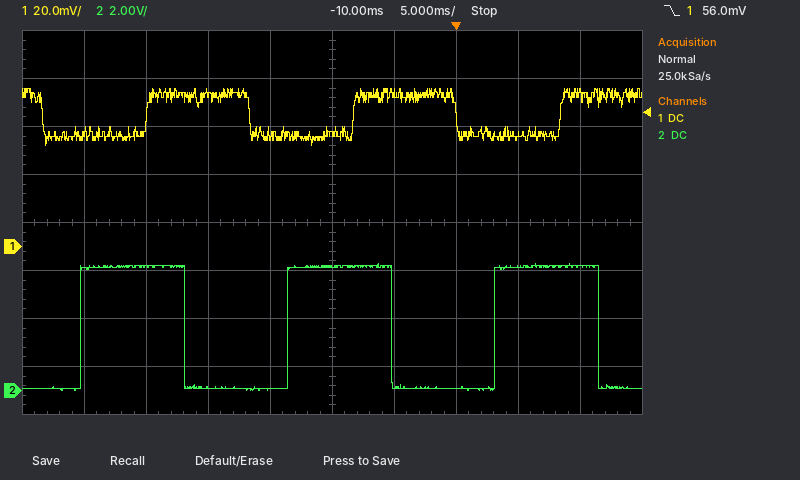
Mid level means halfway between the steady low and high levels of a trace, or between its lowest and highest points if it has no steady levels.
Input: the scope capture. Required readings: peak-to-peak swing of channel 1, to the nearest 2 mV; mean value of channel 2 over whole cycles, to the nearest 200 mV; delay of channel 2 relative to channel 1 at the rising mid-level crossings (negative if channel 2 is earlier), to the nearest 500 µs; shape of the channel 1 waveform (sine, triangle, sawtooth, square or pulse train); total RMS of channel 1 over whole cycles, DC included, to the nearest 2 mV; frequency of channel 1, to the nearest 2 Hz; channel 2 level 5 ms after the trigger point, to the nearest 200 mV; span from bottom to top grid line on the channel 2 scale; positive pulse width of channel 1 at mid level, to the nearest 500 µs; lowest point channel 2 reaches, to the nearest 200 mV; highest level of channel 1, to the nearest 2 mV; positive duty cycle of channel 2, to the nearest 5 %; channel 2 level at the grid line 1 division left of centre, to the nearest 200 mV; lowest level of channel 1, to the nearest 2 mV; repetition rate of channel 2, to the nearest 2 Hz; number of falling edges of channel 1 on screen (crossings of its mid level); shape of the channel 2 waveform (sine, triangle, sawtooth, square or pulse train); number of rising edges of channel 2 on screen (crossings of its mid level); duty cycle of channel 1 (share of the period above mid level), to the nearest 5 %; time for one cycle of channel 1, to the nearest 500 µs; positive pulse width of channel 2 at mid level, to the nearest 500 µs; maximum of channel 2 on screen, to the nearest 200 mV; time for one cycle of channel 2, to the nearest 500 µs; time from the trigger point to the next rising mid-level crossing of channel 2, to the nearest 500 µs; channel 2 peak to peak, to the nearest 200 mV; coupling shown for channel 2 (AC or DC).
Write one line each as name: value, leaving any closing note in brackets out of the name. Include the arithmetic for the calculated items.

peak-to-peak swing of channel 1, to the nearest 2 mV: 66 mV − (42 mV) = 24 mV
mean value of channel 2 over whole cycles, to the nearest 200 mV: 0.0 V + 0.5 × (5.2 V − (0.0 V)) ≈ 2.6 V
delay of channel 2 relative to channel 1 at the rising mid-level crossings (negative if channel 2 is earlier), to the nearest 500 µs: -5.5 ms
shape of the channel 1 waveform: square
total RMS of channel 1 over whole cycles, DC included, to the nearest 2 mV: √(0.5 × (66 mV)² + 0.5 × (46 mV)²) ≈ 56.9 mV, so 56 mV to the nearest 2 mV
frequency of channel 1, to the nearest 2 Hz: 1 / 16.5 ms ≈ 60.6 Hz, so 60 Hz to the nearest 2 Hz
channel 2 level 5 ms after the trigger point, to the nearest 200 mV: 5.2 V
span from bottom to top grid line on the channel 2 scale: 16 V
positive pulse width of channel 1 at mid level, to the nearest 500 µs: 8.5 ms
lowest point channel 2 reaches, to the nearest 200 mV: 0.0 V
highest level of channel 1, to the nearest 2 mV: 66 mV
positive duty cycle of channel 2, to the nearest 5 %: 8.5 ms / 16.5 ms ≈ 51.5 %, so 50 % to the nearest 5 %
channel 2 level at the grid line 1 division left of centre, to the nearest 200 mV: 0.0 V
lowest level of channel 1, to the nearest 2 mV: 42 mV
repetition rate of channel 2, to the nearest 2 Hz: 1 / 16.5 ms ≈ 60.6 Hz, so 60 Hz to the nearest 2 Hz
number of falling edges of channel 1 on screen: 3
shape of the channel 2 waveform: square
number of rising edges of channel 2 on screen: 3
duty cycle of channel 1 (share of the period above mid level), to the nearest 5 %: 8.5 ms / 16.5 ms ≈ 51.5 %, so 50 % to the nearest 5 %
time for one cycle of channel 1, to the nearest 500 µs: 16.5 ms
positive pulse width of channel 2 at mid level, to the nearest 500 µs: 8.5 ms
maximum of channel 2 on screen, to the nearest 200 mV: 5.2 V
time for one cycle of channel 2, to the nearest 500 µs: 16.5 ms
time from the trigger point to the next rising mid-level crossing of channel 2, to the nearest 500 µs: 3.0 ms
channel 2 peak to peak, to the nearest 200 mV: 5.2 V − (0.0 V) = 5.2 V
coupling shown for channel 2: DC
